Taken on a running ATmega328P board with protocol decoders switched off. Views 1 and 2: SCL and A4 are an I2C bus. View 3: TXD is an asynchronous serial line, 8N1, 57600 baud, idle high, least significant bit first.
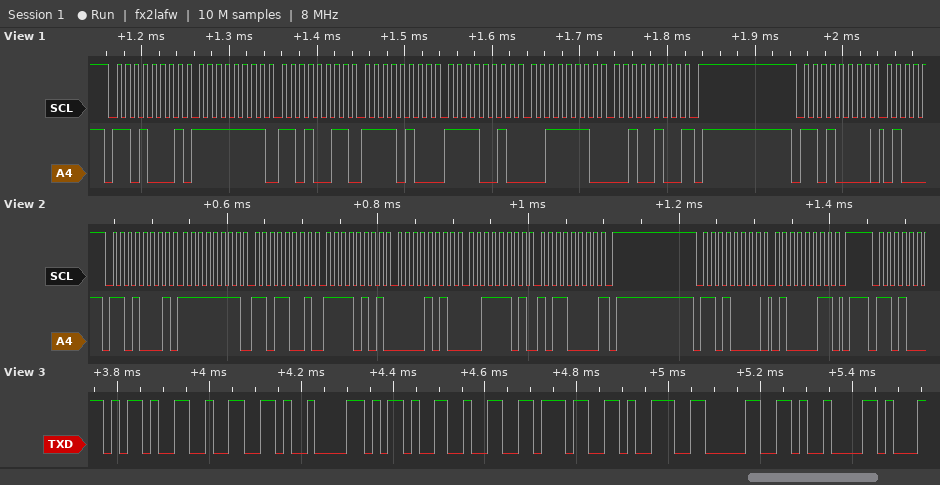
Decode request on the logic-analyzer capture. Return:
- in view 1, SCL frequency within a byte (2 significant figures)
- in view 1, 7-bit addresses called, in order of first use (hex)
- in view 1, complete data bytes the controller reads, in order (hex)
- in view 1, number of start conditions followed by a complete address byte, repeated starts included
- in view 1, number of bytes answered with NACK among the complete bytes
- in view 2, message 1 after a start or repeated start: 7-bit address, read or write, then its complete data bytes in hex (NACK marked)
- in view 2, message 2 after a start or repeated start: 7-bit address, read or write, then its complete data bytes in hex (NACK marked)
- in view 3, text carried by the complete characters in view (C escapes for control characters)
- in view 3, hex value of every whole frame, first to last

100 kHz
0x68
FF D3 F4 F2 3E 24
2
1
0x68 read: FF D9 F5 0A 3D B0 NACK
0x68 write: 43
"-2\t-2790\t"
2D 32 09 2D 32 37 39 30 09
